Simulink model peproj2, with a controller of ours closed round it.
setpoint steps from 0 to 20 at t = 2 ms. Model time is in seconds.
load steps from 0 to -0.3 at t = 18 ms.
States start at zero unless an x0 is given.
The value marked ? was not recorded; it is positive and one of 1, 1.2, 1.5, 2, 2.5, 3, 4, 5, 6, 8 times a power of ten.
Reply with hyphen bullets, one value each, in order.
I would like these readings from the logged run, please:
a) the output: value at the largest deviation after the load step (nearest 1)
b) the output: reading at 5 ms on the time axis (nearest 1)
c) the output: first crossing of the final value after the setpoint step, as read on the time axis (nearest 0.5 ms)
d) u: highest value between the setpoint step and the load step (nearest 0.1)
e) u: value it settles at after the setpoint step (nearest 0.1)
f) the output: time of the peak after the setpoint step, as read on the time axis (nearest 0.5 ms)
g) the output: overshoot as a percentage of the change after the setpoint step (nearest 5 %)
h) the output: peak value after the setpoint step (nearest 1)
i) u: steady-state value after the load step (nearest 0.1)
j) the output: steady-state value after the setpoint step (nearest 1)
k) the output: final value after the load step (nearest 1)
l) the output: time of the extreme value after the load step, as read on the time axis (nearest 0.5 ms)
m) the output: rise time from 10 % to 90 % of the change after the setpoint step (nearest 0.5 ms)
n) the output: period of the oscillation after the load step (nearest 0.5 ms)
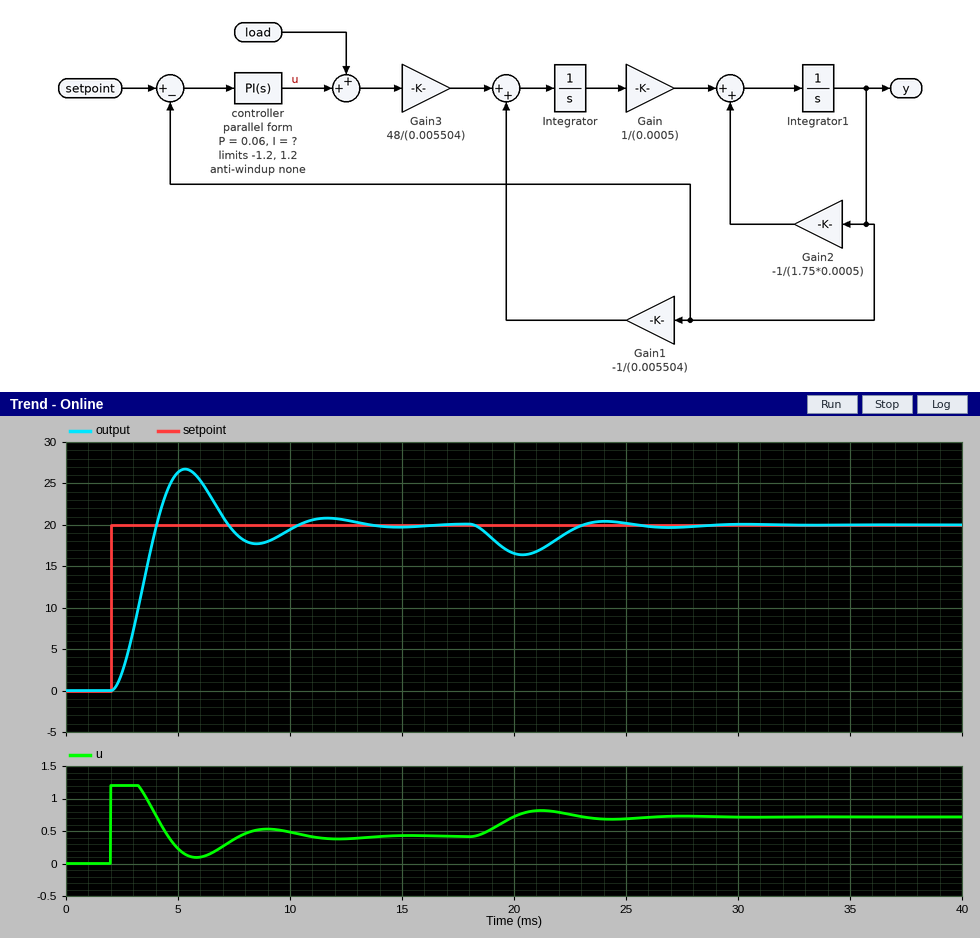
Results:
- 16
- 26
- 4.0 ms
- 1.2
- 0.4
- 5.5 ms
- 35 %
- 27
- 0.7
- 20
- 20
- 20.5 ms
- 1.5 ms
- 6.5 ms
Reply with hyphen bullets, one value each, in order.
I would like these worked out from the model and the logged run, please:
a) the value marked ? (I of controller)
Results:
- 30
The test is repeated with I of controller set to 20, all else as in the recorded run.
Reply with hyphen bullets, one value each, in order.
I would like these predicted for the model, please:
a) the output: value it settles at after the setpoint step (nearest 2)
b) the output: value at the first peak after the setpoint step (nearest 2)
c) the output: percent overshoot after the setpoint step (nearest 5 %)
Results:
- 20
- 24
- 20 %
